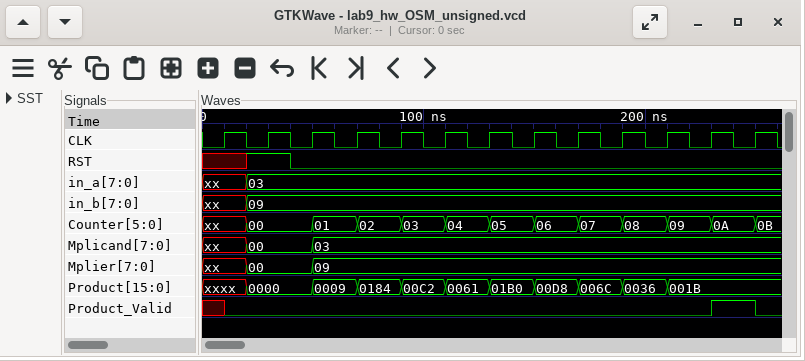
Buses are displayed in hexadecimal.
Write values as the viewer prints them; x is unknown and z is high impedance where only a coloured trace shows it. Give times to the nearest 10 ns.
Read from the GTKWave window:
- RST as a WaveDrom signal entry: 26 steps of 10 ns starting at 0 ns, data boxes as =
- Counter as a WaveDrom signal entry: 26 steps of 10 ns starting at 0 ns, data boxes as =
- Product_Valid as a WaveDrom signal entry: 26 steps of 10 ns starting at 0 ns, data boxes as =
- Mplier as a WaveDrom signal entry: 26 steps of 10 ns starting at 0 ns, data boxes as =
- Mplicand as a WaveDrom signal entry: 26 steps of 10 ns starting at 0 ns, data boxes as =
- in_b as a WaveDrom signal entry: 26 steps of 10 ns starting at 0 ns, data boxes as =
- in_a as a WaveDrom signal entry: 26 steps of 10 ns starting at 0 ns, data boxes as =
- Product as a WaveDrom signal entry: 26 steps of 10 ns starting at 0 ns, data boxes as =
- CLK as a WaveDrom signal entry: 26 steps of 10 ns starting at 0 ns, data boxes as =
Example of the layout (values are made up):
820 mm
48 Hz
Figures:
{name: 'RST', wave: 'x.1.0.....................'}
{name: 'Counter', wave: 'x.=..=.=.=.=.=.=.=.=.=.=.=', data: '00 01 02 03 04 05 06 07 08 09 0A 0B'}
{name: 'Product_Valid', wave: 'x0.....................1.0'}
{name: 'Mplier', wave: 'x.=..=....................', data: '00 09'}
{name: 'Mplicand', wave: 'x.=..=....................', data: '00 03'}
{name: 'in_b', wave: 'x.=.......................', data: '09'}
{name: 'in_a', wave: 'x.=.......................', data: '03'}
{name: 'Product', wave: 'x.=..=.=.=.=.=.=.=.=.=....', data: '0000 0009 0184 00C2 0061 01B0 00D8 006C 0036 001B'}
{name: 'CLK', wave: '01010101010101010101010101'}
